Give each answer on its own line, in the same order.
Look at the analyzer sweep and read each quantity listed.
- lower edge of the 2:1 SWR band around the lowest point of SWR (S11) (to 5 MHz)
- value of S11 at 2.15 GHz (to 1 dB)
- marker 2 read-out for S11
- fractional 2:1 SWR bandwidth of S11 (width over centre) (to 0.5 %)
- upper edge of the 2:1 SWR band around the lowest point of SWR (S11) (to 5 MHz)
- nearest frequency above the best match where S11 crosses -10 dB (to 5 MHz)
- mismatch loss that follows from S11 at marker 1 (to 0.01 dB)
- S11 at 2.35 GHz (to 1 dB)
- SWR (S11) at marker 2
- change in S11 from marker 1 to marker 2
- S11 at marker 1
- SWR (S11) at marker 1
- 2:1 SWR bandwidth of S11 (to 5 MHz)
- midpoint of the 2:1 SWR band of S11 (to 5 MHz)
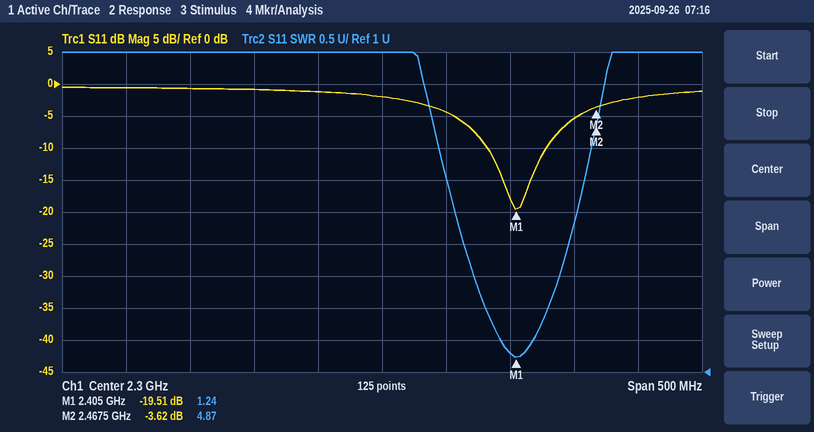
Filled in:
2.380 GHz
-1 dB
-3.62 dB
2.0 %
2.430 GHz
2.430 GHz
0.05 dB
-4 dB
4.87
15.89 dB
-19.51 dB
1.24
50 MHz
2.405 GHz
